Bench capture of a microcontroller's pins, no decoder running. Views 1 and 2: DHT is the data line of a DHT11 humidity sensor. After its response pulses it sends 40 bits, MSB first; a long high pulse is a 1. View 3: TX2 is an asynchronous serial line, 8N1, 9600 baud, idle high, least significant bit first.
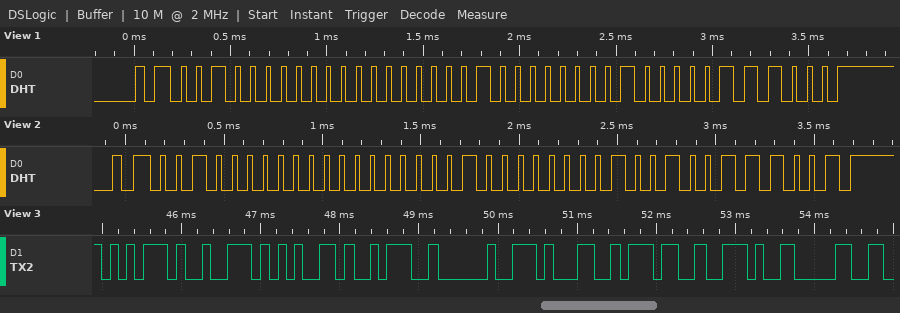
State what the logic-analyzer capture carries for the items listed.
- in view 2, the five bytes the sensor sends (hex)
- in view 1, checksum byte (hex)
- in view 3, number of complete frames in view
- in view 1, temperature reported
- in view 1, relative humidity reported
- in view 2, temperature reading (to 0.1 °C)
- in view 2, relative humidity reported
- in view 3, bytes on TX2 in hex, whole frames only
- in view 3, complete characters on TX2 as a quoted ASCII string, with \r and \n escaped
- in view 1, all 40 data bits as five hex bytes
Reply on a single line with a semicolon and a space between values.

20 00 10 09 39; 0x38; 9; 16.8 °C; 32 %; 16.9 °C; 32 %; 75 72 65 3A 20 31 37 2E 30; "ure: 17.0"; 20 00 10 08 38
